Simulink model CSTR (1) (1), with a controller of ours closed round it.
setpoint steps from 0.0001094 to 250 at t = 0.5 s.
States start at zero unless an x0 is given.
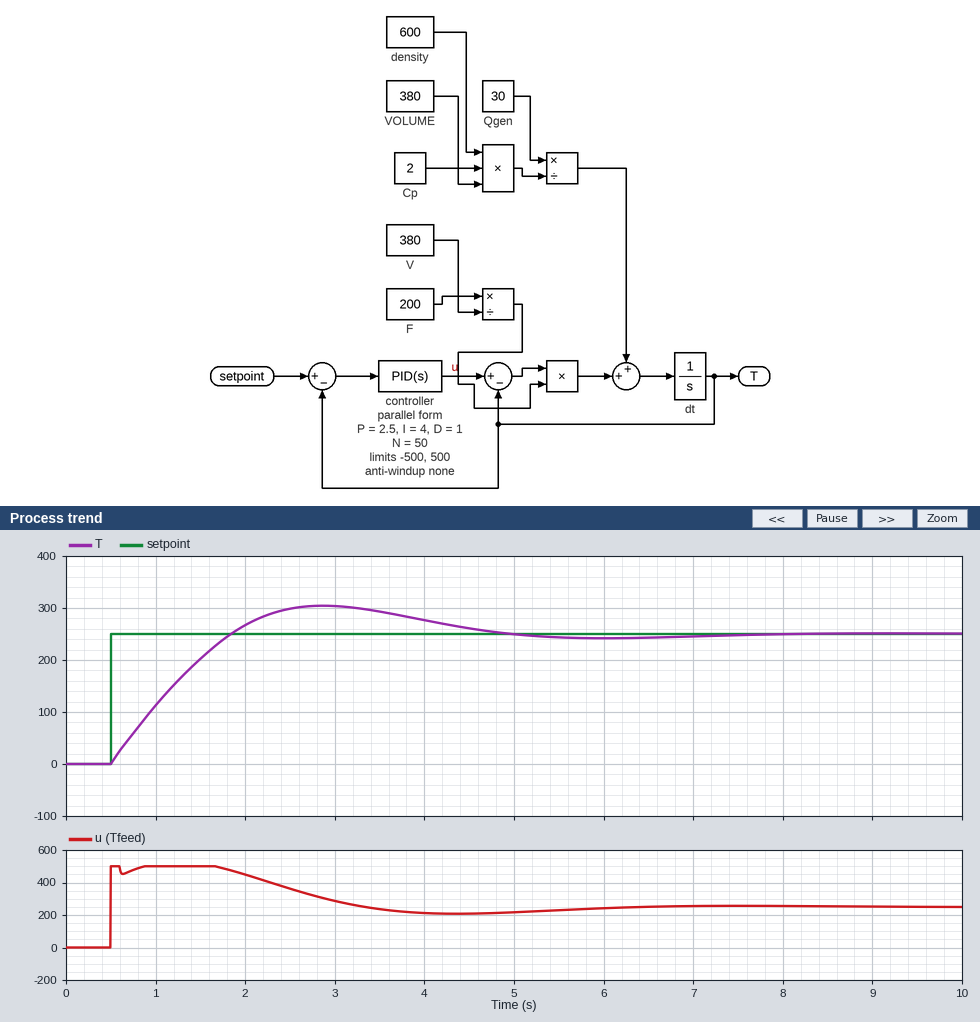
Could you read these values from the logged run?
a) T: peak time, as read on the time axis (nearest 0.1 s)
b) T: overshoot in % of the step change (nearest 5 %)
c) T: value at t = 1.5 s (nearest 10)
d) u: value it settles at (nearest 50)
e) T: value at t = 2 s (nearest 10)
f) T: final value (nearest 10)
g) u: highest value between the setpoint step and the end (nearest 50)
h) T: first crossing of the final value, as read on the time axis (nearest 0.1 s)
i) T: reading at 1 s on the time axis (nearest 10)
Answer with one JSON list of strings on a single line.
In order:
["2.9 s", "20 %", "200", "250", "270", "250", "500", "1.8 s", "110"]
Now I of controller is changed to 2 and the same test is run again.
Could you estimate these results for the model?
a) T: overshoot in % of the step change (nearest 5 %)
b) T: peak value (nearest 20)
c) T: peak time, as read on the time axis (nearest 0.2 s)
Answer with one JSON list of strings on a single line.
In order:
["10 %", "280", "3.8 s"]
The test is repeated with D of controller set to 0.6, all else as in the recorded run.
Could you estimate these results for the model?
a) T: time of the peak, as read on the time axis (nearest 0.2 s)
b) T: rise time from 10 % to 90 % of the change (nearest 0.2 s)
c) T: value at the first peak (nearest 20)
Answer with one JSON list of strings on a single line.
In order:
["2.8 s", "1.0 s", "300"]
